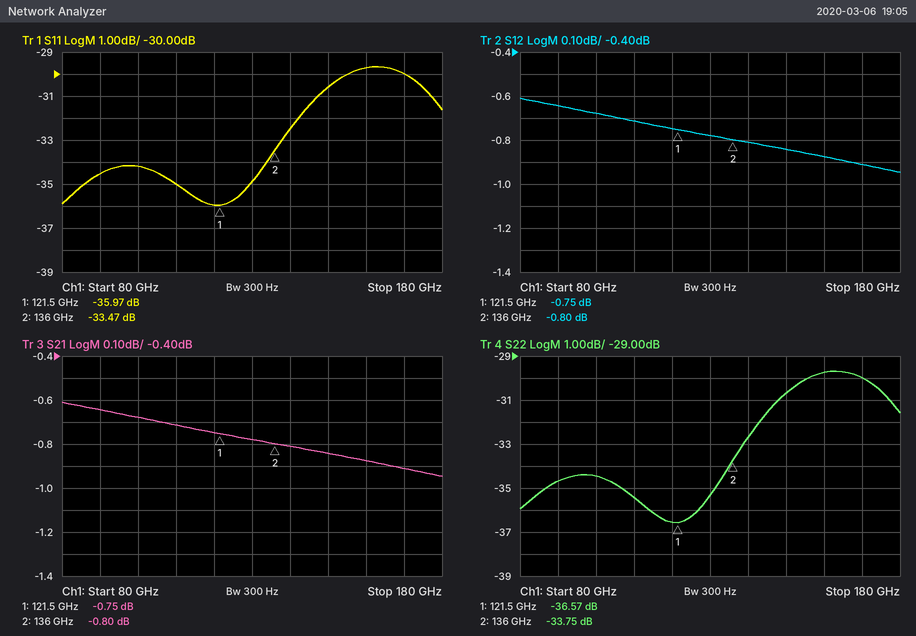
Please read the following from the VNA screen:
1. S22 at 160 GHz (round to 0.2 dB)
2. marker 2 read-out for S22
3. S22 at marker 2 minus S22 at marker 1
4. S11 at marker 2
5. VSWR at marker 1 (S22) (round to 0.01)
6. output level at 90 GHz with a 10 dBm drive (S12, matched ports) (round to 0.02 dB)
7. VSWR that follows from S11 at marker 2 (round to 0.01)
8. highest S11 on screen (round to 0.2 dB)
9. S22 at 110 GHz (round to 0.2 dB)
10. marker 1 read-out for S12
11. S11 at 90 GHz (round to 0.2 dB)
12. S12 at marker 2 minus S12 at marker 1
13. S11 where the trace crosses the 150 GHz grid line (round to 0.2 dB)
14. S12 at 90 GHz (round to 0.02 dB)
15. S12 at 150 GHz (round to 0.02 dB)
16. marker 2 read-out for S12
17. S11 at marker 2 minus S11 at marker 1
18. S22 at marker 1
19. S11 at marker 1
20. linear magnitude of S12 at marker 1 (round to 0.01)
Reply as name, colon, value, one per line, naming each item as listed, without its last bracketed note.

S22 at 160 GHz: -29.8 dB
marker 2 read-out for S22: -33.75 dB
S22 at marker 2 minus S22 at marker 1: 2.82 dB
S11 at marker 2: -33.47 dB
VSWR at marker 1 (S22): 1.03
output level at 90 GHz with a 10 dBm drive (S12, matched ports): 9.36 dBm
VSWR that follows from S11 at marker 2: 1.04
highest S11 on screen: -29.6 dB
S22 at 110 GHz: -35.4 dB
marker 1 read-out for S12: -0.75 dB
S11 at 90 GHz: -34.6 dB
S12 at marker 2 minus S12 at marker 1: -0.05 dB
S11 where the trace crosses the 150 GHz grid line: -30.6 dB
S12 at 90 GHz: -0.64 dB
S12 at 150 GHz: -0.84 dB
marker 2 read-out for S12: -0.80 dB
S11 at marker 2 minus S11 at marker 1: 2.50 dB
S22 at marker 1: -36.57 dB
S11 at marker 1: -35.97 dB
linear magnitude of S12 at marker 1: 0.92
